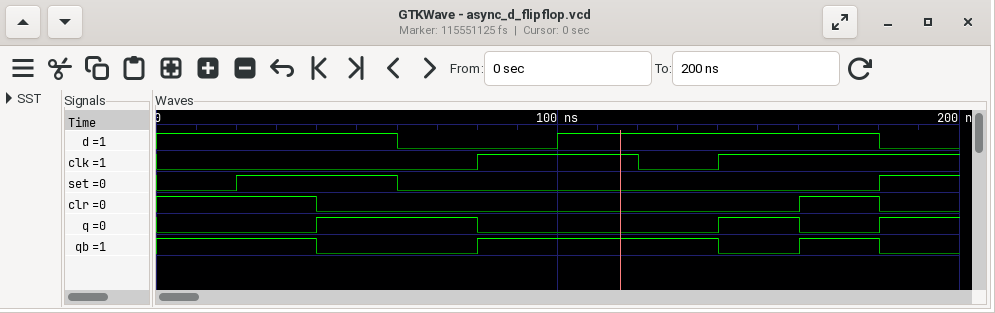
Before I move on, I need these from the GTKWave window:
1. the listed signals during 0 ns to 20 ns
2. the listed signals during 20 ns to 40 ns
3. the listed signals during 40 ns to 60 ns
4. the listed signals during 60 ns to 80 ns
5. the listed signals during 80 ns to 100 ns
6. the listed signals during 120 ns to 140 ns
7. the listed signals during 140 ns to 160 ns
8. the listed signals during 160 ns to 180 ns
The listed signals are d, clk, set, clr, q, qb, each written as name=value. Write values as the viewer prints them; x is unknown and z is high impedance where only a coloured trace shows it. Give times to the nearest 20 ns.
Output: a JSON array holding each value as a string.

["d=1, clk=0, set=0, clr=1, q=0, qb=1", "d=1, clk=0, set=1, clr=1, q=0, qb=1", "d=1, clk=0, set=1, clr=0, q=1, qb=0", "d=0, clk=0, set=0, clr=0, q=1, qb=0", "d=0, clk=1, set=0, clr=0, q=0, qb=1", "d=1, clk=0, set=0, clr=0, q=0, qb=1", "d=1, clk=1, set=0, clr=0, q=1, qb=0", "d=1, clk=1, set=0, clr=1, q=0, qb=1"]
